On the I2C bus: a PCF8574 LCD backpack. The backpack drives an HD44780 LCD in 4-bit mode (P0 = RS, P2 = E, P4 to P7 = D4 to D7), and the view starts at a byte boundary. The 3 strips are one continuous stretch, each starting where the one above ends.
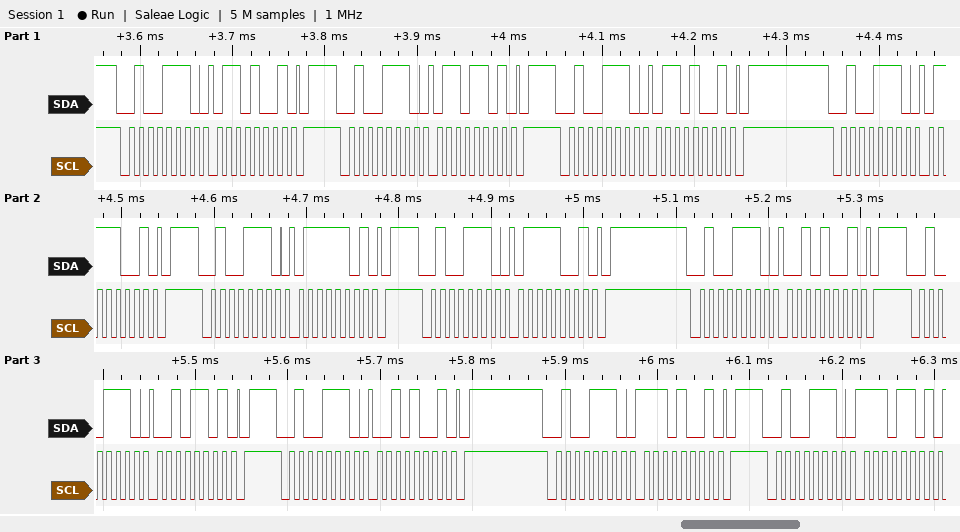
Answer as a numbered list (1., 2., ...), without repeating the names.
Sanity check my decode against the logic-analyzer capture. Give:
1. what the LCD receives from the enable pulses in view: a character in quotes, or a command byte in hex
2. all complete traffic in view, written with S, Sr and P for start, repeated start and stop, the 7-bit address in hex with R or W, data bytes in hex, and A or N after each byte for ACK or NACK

1. 'g'
2. S 27W A 69 A P S 27W A 6D A P S 27W A 69 A P S 27W A 79 A P S 27W A 7D A P S 27W A 79 A P S 27W A 29 A P S 27W A 2D A P S 27W A 29 A P S 27W A E9 A P S 27W A ED A
